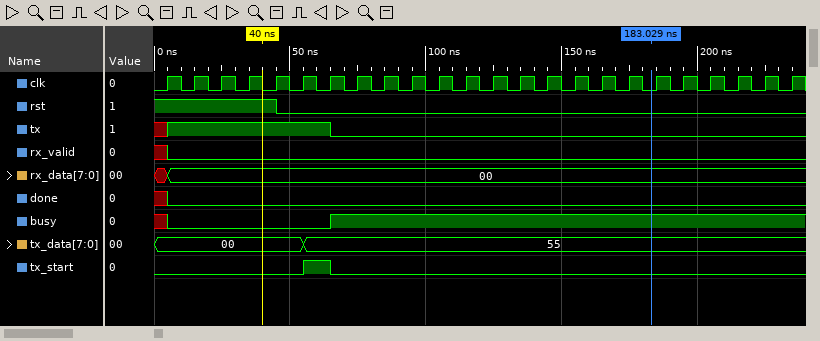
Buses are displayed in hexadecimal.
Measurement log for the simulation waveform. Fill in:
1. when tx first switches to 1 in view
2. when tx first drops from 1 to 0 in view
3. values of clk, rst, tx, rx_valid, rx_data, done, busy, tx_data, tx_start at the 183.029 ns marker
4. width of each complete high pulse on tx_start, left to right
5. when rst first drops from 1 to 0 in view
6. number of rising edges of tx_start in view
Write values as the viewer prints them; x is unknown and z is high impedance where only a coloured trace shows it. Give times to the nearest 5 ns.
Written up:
5 ns
65 ns
clk=0, rst=0, tx=0, rx_valid=0, rx_data=00, done=0, busy=1, tx_data=55, tx_start=0
10 ns
45 ns
1
